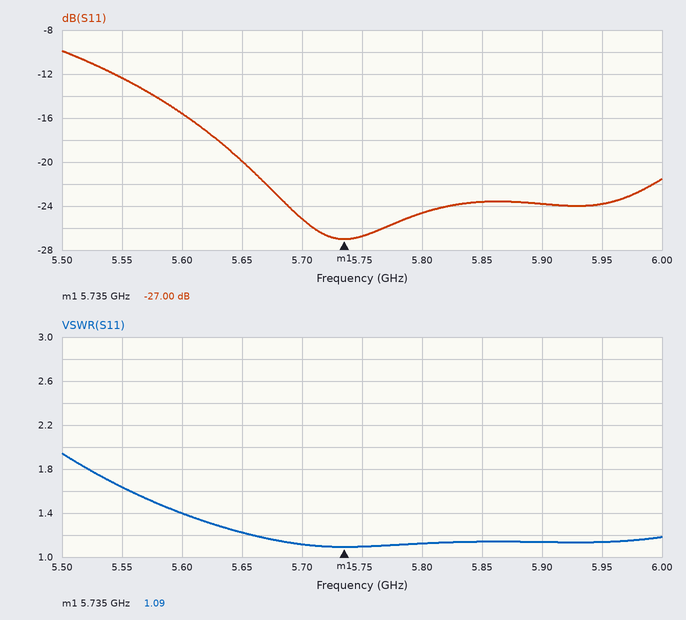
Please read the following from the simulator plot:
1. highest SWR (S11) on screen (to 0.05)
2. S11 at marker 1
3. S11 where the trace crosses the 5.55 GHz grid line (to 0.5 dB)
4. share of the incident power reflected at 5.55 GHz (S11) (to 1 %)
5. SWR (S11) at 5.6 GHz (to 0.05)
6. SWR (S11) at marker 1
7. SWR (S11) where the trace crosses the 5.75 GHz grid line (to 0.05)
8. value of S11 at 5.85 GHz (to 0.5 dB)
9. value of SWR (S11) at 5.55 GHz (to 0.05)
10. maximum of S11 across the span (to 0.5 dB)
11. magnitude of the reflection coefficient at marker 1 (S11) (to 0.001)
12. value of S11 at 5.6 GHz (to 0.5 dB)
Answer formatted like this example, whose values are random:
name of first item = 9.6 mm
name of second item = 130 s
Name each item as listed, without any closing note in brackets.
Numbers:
highest SWR (S11) on screen = 1.95
S11 at marker 1 = -27.00 dB
S11 where the trace crosses the 5.55 GHz grid line = -12.5 dB
share of the incident power reflected at 5.55 GHz (S11) = 6 %
SWR (S11) at 5.6 GHz = 1.40
SWR (S11) at marker 1 = 1.09
SWR (S11) where the trace crosses the 5.75 GHz grid line = 1.10
value of S11 at 5.85 GHz = -23.5 dB
value of SWR (S11) at 5.55 GHz = 1.65
maximum of S11 across the span = -10.0 dB
magnitude of the reflection coefficient at marker 1 (S11) = 0.045
value of S11 at 5.6 GHz = -15.5 dB
